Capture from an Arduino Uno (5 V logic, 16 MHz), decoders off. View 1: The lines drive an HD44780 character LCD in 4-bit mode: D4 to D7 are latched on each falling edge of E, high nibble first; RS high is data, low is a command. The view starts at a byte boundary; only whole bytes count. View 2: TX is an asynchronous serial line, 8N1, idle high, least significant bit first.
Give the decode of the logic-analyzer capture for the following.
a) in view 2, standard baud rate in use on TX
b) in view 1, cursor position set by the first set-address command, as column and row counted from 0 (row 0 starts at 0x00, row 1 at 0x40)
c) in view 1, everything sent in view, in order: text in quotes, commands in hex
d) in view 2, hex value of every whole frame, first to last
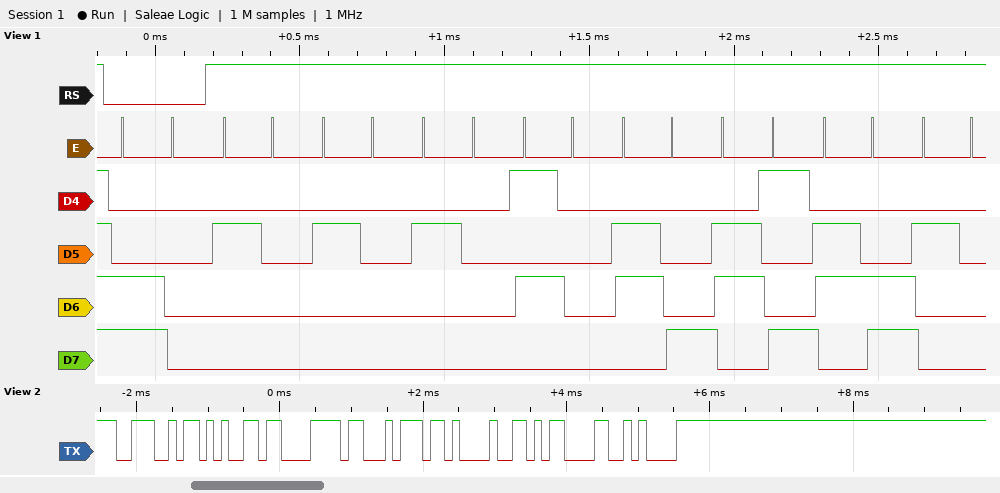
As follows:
9600 baud
column 0, row 1
0xC0 "   Phil "
4E 65 78 74 21 0D 0A
